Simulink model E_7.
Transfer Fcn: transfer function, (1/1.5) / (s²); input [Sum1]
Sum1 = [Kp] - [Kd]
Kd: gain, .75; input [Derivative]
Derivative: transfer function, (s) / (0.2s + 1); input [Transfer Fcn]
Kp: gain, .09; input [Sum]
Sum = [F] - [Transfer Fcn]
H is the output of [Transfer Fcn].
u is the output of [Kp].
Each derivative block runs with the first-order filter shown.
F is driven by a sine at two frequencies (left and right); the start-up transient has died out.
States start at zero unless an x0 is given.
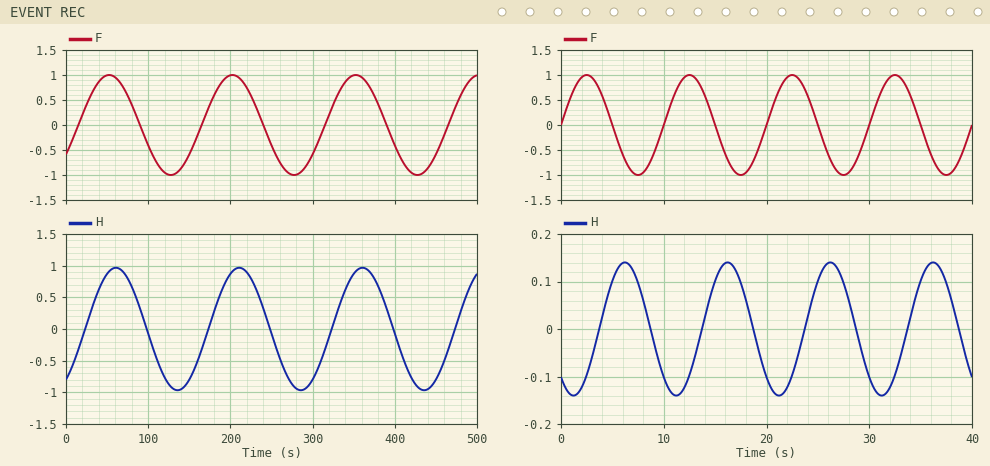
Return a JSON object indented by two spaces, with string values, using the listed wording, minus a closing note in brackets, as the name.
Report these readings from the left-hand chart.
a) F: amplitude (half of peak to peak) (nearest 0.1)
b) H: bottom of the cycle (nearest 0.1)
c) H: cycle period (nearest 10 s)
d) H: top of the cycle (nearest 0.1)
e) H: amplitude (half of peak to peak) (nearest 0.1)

{
  "F: amplitude (half of peak to peak)": "1.0",
  "H: bottom of the cycle": "-1.0",
  "H: cycle period": "150 s",
  "H: top of the cycle": "1.0",
  "H: amplitude (half of peak to peak)": "1.0"
}
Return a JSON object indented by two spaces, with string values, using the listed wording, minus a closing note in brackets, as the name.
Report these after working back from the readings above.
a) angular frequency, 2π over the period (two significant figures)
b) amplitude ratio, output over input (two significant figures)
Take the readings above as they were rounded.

{
  "angular frequency, 2π over the period": "0.042 rad/s",
  "amplitude ratio, output over input": "1.0"
}
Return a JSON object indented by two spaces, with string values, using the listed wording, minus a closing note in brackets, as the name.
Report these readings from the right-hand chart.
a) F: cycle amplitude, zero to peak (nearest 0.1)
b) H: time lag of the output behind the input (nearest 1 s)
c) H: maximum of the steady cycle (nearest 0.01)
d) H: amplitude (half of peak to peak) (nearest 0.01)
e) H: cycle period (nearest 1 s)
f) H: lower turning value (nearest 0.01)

{
  "F: cycle amplitude, zero to peak": "1.0",
  "H: time lag of the output behind the input": "4 s",
  "H: maximum of the steady cycle": "0.14",
  "H: amplitude (half of peak to peak)": "0.14",
  "H: cycle period": "10 s",
  "H: lower turning value": "-0.14"
}
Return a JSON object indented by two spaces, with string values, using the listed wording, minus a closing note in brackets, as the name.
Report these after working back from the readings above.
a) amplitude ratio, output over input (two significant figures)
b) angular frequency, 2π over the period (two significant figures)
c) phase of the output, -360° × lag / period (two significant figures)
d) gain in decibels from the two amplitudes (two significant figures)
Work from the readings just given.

{
  "amplitude ratio, output over input": "0.14",
  "angular frequency, 2π over the period": "0.63 rad/s",
  "phase of the output, -360° × lag / period": "-140°",
  "gain in decibels from the two amplitudes": "-17 dB"
}
